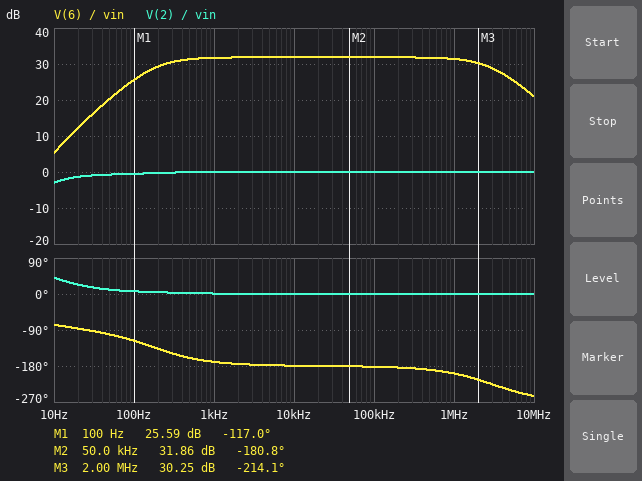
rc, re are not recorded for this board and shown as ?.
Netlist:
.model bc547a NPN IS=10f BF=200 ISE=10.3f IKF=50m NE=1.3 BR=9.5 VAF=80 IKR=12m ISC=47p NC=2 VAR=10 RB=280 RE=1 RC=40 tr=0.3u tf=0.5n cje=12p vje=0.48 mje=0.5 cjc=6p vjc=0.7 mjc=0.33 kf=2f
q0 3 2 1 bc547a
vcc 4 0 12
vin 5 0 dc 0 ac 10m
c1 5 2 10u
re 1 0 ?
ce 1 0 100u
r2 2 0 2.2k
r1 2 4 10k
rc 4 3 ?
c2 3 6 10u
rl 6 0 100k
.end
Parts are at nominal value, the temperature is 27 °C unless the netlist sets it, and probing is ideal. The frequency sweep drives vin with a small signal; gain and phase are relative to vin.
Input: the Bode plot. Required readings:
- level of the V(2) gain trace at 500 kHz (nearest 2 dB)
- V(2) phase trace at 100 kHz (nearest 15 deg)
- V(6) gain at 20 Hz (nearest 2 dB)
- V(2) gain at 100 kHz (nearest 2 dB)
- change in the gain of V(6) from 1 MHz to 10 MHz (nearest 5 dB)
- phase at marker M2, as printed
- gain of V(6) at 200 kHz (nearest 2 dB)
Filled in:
0 dB
0 deg
12 dB
0 dB
-10 dB
-180.8 deg
32 dB
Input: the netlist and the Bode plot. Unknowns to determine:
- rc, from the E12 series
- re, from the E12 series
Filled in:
390 Ω
330 Ω
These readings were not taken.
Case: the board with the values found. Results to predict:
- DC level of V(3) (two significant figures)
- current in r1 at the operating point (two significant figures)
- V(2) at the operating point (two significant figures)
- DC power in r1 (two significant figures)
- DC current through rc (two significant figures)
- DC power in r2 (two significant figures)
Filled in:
10 V
990 µA
2.1 V
9.8 mW
4.2 mA
2.0 mW
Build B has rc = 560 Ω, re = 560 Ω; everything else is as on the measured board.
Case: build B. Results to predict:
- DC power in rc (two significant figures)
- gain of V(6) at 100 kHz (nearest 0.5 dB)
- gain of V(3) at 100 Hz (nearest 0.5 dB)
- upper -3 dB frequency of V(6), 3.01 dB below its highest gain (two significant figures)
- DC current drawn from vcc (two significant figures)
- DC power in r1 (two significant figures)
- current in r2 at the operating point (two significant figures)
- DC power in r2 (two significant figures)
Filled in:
3.7 mW
32.0 dB
28.0 dB
3.2 MHz
3.5 mA
9.7 mW
970 µA
2.1 mW
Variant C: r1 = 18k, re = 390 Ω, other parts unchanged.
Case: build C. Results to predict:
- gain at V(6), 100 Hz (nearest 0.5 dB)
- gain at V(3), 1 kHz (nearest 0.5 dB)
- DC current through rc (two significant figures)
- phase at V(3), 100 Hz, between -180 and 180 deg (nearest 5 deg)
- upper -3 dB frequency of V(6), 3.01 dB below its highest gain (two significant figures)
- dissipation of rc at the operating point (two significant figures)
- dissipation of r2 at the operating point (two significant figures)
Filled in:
23.0 dB
25.5 dB
1.6 mA
-135 deg
5.3 MHz
950 µW
750 µW
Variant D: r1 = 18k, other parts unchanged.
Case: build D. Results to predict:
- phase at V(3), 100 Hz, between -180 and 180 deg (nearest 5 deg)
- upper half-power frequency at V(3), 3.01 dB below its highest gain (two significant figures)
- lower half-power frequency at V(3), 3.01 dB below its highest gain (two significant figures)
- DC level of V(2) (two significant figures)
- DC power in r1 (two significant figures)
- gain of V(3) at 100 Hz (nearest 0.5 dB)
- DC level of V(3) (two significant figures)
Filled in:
-135 deg
4.8 MHz
100 Hz
1.3 V
6.4 mW
23.5 dB
11 V
